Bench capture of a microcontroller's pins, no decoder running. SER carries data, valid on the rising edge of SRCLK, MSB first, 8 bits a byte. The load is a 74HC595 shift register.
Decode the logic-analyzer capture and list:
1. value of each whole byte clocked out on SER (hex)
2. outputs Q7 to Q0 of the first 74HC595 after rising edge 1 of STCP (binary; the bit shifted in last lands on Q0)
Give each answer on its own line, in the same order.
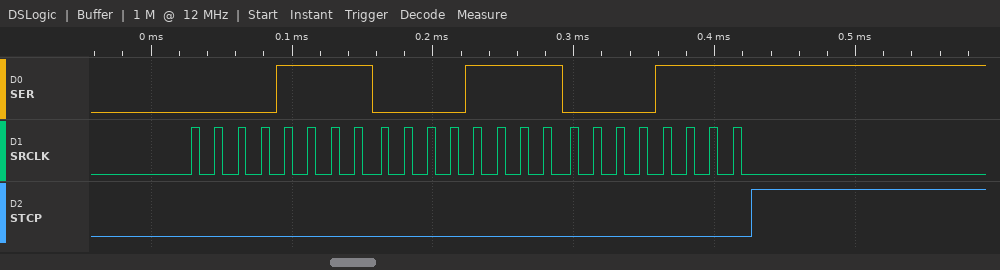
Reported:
0F 0F 0F
00001111
